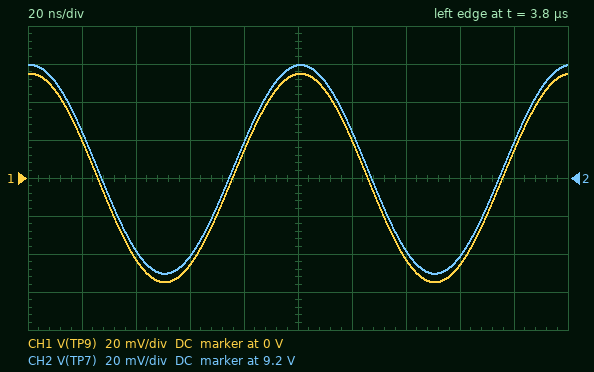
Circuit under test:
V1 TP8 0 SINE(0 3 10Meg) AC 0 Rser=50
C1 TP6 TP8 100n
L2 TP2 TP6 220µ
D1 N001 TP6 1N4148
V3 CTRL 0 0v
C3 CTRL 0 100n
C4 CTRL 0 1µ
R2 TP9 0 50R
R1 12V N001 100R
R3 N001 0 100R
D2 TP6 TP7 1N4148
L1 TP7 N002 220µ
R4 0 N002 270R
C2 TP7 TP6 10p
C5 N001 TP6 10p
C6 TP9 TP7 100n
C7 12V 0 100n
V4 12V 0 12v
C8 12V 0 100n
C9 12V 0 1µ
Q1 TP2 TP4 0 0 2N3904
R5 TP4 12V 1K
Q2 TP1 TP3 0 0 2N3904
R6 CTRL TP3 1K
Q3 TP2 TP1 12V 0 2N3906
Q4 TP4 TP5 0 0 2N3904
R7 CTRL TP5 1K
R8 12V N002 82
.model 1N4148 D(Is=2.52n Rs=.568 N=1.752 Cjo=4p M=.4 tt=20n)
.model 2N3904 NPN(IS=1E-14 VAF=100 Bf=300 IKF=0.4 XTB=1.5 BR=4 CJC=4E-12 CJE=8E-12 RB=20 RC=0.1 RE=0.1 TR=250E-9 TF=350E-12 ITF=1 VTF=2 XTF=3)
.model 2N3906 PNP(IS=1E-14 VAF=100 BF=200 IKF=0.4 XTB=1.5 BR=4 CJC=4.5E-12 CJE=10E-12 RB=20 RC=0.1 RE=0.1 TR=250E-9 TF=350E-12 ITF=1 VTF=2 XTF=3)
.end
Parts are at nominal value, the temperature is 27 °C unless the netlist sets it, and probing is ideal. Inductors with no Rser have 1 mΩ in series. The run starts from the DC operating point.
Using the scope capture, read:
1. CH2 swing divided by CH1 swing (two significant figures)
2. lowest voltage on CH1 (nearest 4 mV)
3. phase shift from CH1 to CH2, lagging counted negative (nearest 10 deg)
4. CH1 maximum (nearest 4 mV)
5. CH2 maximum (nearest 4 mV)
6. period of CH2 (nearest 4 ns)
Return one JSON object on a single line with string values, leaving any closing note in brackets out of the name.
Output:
{"CH2 swing divided by CH1 swing": "1.0", "lowest voltage on CH1": "-56 mV", "phase shift from CH1 to CH2, lagging counted negative": "0 deg", "CH1 maximum": "56 mV", "CH2 maximum": "9.260 V", "period of CH2": "100 ns"}
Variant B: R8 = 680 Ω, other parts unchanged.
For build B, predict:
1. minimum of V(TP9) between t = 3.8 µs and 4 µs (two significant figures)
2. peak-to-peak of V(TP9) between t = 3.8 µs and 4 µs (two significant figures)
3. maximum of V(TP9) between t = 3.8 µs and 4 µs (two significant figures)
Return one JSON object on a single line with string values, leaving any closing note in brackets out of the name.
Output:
{"minimum of V(TP9) between t = 3.8 µs and 4 µs": "-58 mV", "peak-to-peak of V(TP9) between t = 3.8 µs and 4 µs": "120 mV", "maximum of V(TP9) between t = 3.8 µs and 4 µs": "58 mV"}
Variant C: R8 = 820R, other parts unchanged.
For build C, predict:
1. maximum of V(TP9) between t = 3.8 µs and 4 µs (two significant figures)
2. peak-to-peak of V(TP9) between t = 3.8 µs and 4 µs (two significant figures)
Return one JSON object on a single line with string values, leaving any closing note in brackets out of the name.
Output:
{"maximum of V(TP9) between t = 3.8 µs and 4 µs": "58 mV", "peak-to-peak of V(TP9) between t = 3.8 µs and 4 µs": "120 mV"}
